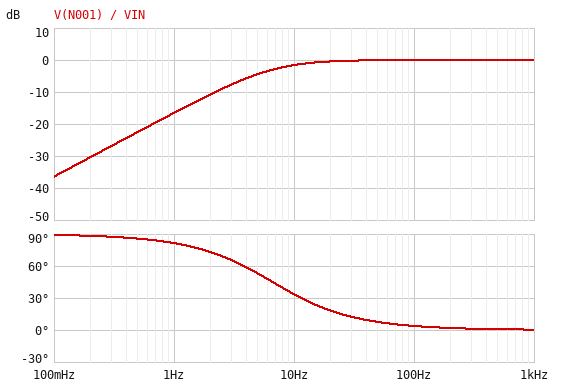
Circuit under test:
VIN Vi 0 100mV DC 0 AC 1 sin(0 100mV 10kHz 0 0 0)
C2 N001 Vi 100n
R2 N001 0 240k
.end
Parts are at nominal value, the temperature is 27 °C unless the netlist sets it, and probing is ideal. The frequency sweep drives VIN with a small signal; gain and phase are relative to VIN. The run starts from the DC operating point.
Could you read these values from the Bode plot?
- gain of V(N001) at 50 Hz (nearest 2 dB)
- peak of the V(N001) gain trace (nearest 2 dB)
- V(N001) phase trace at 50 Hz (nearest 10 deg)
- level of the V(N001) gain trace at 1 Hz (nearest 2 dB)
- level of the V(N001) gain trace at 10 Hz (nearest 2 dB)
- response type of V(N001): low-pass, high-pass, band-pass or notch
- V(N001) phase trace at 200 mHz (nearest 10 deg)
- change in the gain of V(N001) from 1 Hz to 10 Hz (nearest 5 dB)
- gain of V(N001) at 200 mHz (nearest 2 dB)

0 dB
0 dB
10 deg
-16 dB
-2 dB
high-pass
90 deg
15 dB
-30 dB
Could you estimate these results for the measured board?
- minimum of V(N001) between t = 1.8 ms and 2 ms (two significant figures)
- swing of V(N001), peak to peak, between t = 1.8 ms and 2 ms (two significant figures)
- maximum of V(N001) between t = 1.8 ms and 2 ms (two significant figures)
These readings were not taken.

-100 mV
200 mV
100 mV
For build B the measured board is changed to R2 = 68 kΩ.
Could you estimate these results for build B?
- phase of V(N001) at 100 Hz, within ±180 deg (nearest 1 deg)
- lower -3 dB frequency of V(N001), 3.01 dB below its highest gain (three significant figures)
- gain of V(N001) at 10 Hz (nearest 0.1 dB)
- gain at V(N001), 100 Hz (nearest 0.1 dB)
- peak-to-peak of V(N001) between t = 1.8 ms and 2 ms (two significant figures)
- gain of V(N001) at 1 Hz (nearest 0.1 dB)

13 deg
23.4 Hz
-8.1 dB
-0.2 dB
200 mV
-27.4 dB
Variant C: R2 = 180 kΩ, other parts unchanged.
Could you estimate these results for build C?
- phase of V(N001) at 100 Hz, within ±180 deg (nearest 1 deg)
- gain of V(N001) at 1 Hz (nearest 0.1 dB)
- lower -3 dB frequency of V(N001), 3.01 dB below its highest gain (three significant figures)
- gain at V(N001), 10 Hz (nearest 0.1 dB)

5 deg
-19.0 dB
8.84 Hz
-2.5 dB
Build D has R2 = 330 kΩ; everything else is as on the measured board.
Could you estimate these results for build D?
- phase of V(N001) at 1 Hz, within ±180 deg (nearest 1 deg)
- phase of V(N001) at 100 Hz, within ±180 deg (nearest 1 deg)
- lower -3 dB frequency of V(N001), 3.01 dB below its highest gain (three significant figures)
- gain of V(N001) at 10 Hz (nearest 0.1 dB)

78 deg
3 deg
4.82 Hz
-0.9 dB
